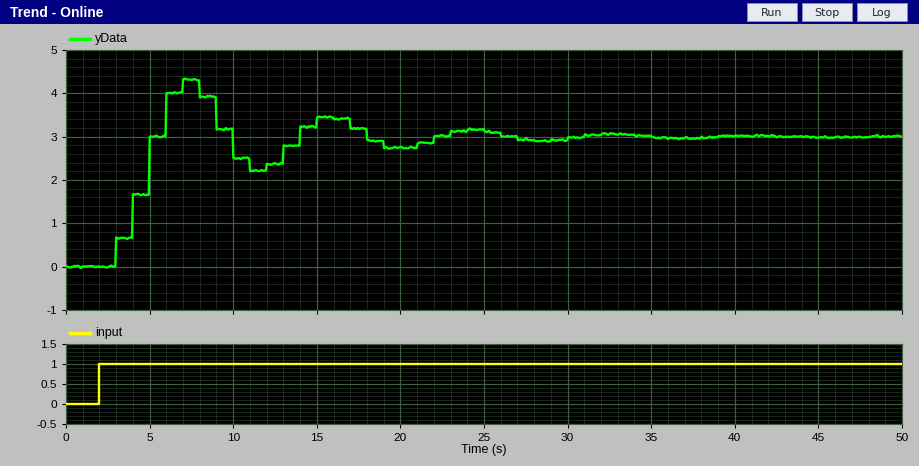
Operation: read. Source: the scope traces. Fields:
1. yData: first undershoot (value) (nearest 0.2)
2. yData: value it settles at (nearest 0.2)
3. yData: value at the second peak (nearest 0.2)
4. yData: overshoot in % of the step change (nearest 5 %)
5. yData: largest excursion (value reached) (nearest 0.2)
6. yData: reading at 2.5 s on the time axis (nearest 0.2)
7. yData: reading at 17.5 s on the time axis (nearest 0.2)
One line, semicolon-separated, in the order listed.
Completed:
2.2; 3.0; 3.4; 45 %; 4.4; 0.0; 3.2
